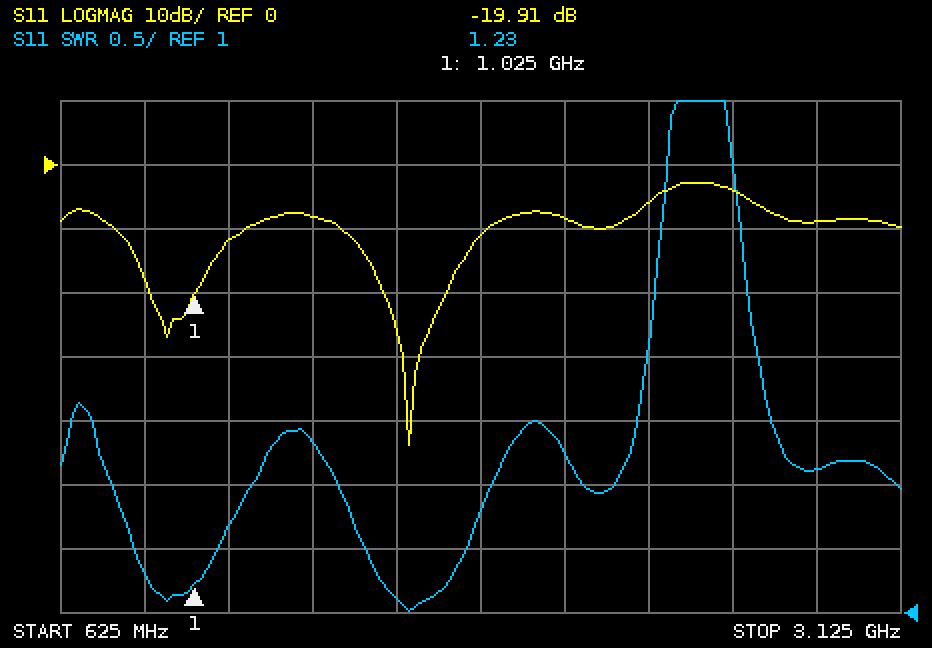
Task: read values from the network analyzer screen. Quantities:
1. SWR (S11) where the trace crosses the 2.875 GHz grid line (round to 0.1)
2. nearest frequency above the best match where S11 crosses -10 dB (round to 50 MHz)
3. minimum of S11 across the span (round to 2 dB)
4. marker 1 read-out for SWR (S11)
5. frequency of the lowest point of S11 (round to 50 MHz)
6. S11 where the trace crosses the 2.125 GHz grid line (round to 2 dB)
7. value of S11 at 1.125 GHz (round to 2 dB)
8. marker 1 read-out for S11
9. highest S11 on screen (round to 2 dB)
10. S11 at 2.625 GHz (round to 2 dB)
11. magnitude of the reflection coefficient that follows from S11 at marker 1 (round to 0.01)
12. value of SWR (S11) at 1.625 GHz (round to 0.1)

2.1
1.90 GHz
-44 dB
1.23
1.65 GHz
-8 dB
-12 dB
-19.91 dB
-2 dB
-4 dB
0.10
1.1
